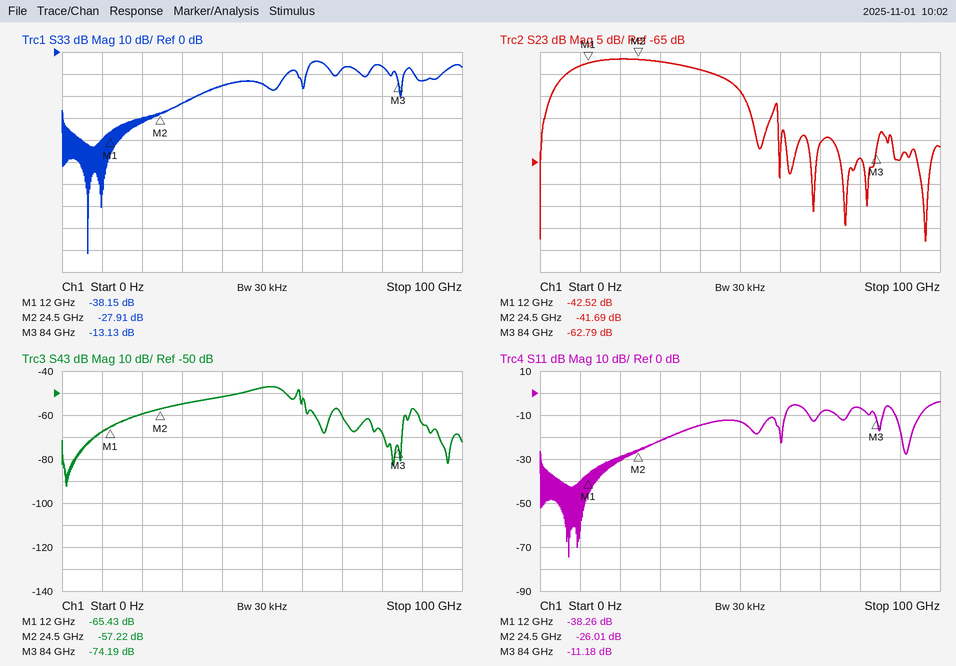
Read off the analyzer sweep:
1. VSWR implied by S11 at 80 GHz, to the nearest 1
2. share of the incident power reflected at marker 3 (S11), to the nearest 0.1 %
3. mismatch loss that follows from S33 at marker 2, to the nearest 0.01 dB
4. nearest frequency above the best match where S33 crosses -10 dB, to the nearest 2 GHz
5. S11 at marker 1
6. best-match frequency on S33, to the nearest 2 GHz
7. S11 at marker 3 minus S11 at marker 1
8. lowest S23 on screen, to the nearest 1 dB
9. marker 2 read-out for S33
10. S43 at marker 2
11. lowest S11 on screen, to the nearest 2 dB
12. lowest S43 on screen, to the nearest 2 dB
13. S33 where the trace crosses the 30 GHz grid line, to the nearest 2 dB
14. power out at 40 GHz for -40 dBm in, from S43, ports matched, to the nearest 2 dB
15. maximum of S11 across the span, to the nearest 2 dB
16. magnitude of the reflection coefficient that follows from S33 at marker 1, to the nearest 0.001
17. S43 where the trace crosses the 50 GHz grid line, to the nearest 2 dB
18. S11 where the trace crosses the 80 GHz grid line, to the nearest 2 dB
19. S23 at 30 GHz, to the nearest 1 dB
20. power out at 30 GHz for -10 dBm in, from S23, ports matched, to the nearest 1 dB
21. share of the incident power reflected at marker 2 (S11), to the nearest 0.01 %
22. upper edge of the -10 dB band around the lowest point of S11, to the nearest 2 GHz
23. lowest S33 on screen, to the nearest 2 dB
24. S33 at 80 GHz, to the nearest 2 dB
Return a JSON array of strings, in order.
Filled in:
["3", "7.6 %", "0.01 dB", "56 GHz", "-38.26 dB", "6 GHz", "27.08 dB", "-83 dB", "-27.91 dB", "-57.22 dB", "-74 dB", "-92 dB", "-24 dB", "-92 dBm", "-4 dB", "0.012", "-48 dB", "-6 dB", "-42 dB", "-52 dBm", "0.25 %", "62 GHz", "-92 dB", "-6 dB"]
